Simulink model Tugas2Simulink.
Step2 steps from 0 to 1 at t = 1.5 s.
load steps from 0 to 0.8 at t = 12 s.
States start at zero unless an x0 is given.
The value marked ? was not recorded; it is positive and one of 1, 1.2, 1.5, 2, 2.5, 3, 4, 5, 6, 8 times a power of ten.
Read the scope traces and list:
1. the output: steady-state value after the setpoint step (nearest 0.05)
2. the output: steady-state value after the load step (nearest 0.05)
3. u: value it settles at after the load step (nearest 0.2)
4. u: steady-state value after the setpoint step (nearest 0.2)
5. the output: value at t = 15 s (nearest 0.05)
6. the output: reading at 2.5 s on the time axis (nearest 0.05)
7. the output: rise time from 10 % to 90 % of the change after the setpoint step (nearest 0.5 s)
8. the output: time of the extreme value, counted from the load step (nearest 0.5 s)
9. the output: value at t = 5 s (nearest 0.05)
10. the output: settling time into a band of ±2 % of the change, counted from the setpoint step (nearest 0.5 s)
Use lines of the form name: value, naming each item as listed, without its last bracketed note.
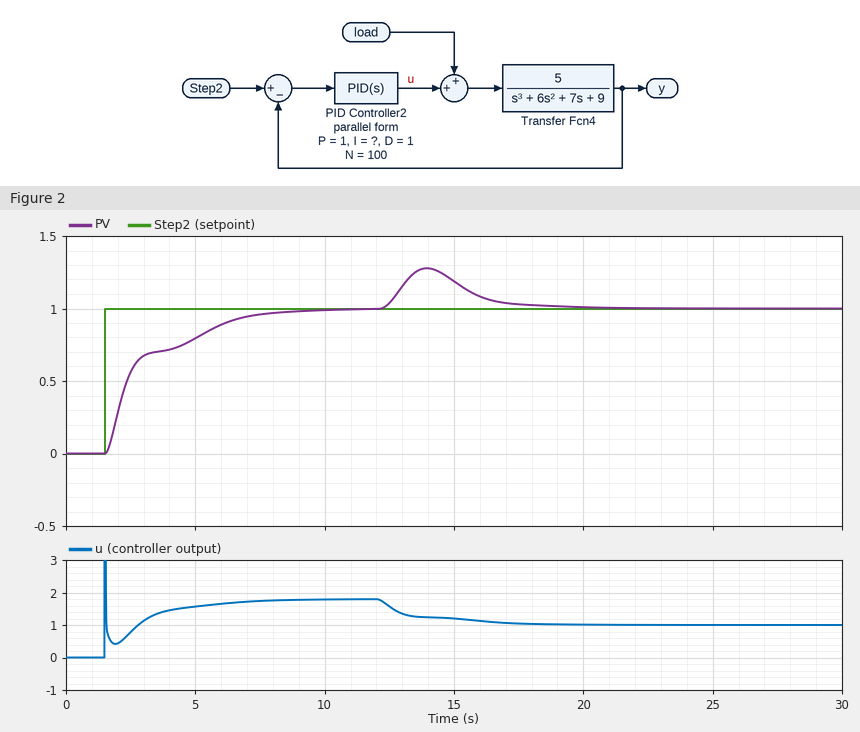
the output: steady-state value after the setpoint step: 1.00
the output: steady-state value after the load step: 1.00
u: value it settles at after the load step: 1.0
u: steady-state value after the setpoint step: 1.8
the output: value at t = 15 s: 1.20
the output: reading at 2.5 s on the time axis: 0.55
the output: rise time from 10 % to 90 % of the change after the setpoint step: 4.5 s
the output: time of the extreme value, counted from the load step: 2.0 s
the output: value at t = 5 s: 0.80
the output: settling time into a band of ±2 % of the change, counted from the setpoint step: 7.5 s
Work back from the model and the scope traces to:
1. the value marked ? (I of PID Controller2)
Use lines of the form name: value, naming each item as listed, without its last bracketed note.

the value marked ?: 1
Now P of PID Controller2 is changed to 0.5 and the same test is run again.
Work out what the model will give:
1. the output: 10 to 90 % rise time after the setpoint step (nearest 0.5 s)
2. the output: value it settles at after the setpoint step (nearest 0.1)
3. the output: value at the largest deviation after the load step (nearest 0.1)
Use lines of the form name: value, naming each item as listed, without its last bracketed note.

the output: 10 to 90 % rise time after the setpoint step: 4.0 s
the output: value it settles at after the setpoint step: 1.0
the output: value at the largest deviation after the load step: 1.3
